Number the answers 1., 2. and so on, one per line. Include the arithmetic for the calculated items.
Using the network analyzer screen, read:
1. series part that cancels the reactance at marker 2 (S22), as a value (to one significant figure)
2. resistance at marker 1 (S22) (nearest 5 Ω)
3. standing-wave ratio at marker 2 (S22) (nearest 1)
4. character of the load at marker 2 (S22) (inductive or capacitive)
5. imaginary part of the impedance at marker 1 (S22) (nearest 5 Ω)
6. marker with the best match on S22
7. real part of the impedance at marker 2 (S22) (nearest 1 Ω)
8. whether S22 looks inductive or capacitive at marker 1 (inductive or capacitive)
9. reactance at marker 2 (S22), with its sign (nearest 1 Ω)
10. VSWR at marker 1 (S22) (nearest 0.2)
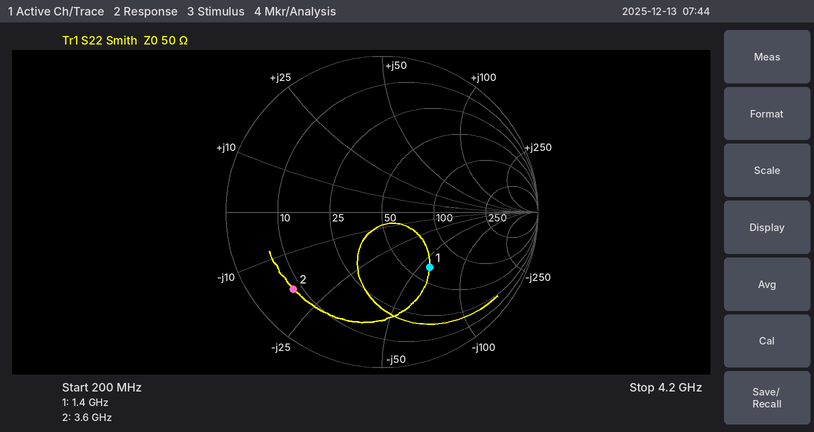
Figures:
1. L = 18 Ω/(2π × 3.6 GHz) ≈ 796 pH, so 800 pH to one significant figure
2. 65 Ω
3. 7
4. capacitive
5. -60 Ω
6. marker 1
7. 8 Ω
8. capacitive
9. -18 Ω
10. 2.8
